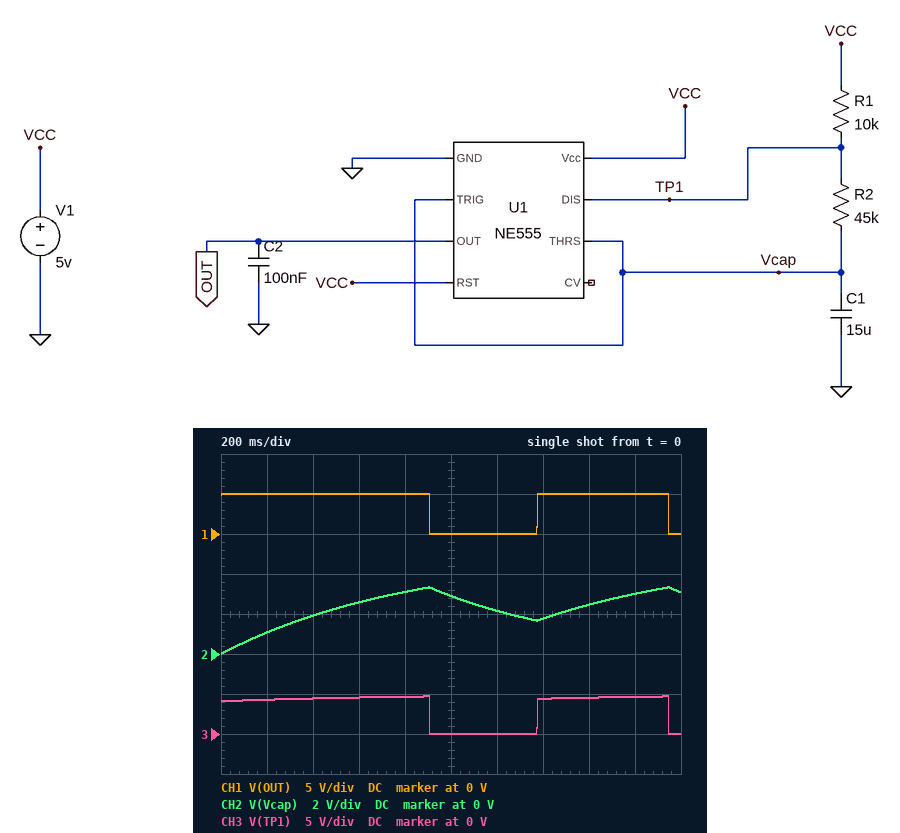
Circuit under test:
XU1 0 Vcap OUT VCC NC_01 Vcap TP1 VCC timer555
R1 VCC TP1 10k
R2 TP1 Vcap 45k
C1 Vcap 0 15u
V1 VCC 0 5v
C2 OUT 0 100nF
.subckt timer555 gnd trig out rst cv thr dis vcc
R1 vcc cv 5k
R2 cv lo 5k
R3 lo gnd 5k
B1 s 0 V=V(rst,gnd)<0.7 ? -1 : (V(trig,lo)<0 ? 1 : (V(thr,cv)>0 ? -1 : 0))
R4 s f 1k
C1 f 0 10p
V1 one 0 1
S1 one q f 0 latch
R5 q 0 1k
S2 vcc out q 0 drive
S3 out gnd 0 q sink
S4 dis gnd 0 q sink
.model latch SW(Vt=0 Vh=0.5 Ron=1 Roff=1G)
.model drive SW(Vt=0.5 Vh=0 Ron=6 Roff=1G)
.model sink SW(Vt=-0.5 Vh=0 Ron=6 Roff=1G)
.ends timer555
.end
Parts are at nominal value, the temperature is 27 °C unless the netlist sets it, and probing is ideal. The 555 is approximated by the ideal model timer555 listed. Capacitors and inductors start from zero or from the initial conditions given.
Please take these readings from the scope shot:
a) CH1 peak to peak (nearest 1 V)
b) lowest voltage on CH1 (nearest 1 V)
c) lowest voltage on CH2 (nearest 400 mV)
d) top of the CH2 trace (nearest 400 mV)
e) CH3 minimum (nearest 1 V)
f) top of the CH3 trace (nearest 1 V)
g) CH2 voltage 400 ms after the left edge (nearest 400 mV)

5 V
0 V
0 V
3.2 V
0 V
5 V
2.0 V
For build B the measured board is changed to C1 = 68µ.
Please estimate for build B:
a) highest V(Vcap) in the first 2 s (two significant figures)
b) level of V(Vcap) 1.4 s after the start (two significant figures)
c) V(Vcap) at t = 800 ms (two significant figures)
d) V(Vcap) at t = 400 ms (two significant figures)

2.1 V
1.6 V
960 mV
510 mV
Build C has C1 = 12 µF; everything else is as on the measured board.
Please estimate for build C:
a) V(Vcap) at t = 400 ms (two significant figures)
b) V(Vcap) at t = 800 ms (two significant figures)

2.3 V
2.9 V
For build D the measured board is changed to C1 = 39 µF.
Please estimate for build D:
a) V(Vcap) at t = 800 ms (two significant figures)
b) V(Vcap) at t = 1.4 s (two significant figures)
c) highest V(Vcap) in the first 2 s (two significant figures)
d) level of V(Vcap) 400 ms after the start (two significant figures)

1.6 V
2.4 V
3.0 V
850 mV
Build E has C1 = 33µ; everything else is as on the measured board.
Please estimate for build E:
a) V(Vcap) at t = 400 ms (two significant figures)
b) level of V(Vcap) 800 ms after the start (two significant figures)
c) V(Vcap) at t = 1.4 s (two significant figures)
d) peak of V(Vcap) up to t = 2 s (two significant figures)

990 mV
1.8 V
2.7 V
3.3 V
